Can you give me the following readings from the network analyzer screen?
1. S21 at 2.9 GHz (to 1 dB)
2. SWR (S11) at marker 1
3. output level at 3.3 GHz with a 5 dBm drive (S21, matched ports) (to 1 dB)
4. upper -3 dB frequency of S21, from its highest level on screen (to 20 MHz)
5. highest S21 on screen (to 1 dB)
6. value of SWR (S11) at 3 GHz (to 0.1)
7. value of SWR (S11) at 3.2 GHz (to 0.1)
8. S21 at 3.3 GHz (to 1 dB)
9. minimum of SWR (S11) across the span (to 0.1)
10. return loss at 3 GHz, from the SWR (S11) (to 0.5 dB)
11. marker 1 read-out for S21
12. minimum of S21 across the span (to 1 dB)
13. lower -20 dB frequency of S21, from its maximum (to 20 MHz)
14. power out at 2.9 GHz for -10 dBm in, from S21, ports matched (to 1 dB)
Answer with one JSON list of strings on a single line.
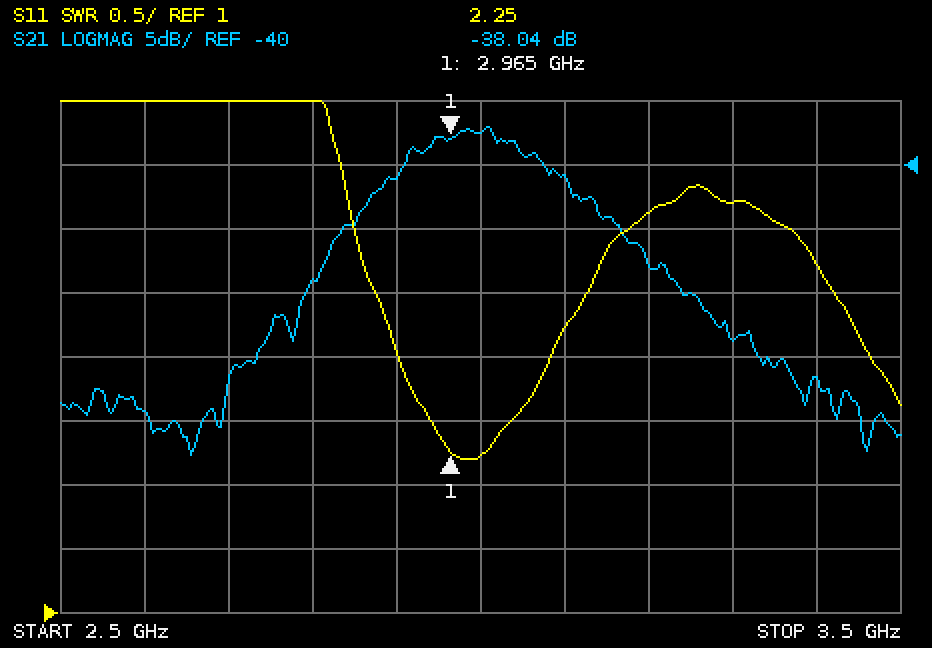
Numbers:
["-41 dB", "2.25", "-49 dBm", "3.08 GHz", "-37 dB", "2.2", "4.1", "-54 dB", "2.2", "8.5 dB", "-38.04 dB", "-63 dB", "2.70 GHz", "-51 dBm"]
